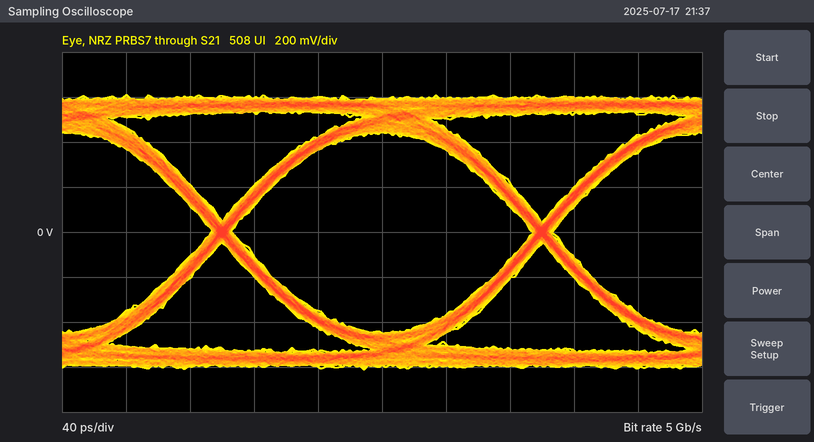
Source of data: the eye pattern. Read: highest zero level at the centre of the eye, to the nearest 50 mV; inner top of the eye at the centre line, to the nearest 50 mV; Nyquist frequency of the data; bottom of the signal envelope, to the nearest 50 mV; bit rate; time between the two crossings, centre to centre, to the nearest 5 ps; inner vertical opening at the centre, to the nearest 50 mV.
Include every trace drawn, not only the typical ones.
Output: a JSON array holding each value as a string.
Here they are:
["-450 mV", "450 mV", "2.5 GHz", "-600 mV", "5 Gb/s", "200 ps", "900 mV"]
